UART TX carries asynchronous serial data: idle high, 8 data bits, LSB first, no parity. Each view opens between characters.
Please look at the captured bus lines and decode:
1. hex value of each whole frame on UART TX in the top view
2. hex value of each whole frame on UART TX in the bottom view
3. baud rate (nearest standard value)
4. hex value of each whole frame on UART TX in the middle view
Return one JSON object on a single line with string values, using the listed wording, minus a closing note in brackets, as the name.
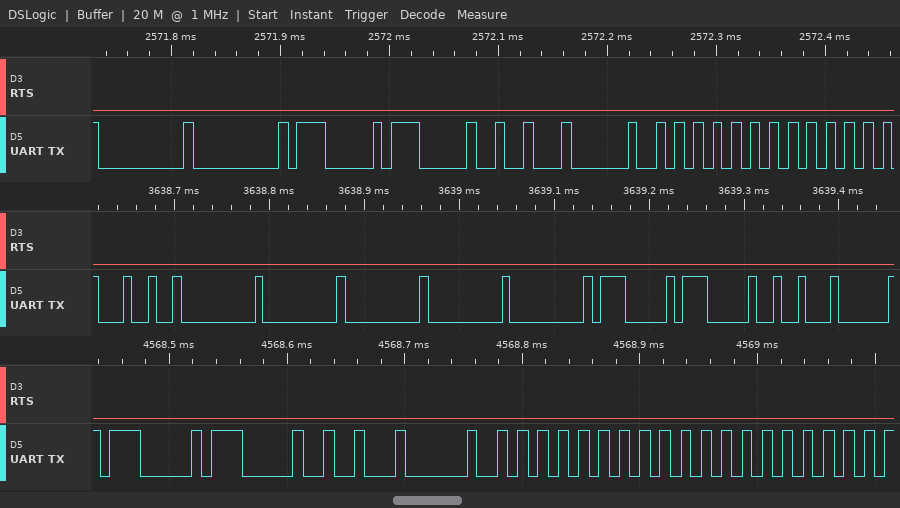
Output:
{"hex value of each whole frame on UART TX in the top view": "00, 00, 07, 07, 12, 20, 55, 55", "hex value of each whole frame on UART TX in the bottom view": "07, 07, 12, 20, 55, 55, 55", "baud rate": "115200 baud", "hex value of each whole frame on UART TX in the middle view": "24, 00, 00, 00, 00, 00, 07, 07, 12"}
